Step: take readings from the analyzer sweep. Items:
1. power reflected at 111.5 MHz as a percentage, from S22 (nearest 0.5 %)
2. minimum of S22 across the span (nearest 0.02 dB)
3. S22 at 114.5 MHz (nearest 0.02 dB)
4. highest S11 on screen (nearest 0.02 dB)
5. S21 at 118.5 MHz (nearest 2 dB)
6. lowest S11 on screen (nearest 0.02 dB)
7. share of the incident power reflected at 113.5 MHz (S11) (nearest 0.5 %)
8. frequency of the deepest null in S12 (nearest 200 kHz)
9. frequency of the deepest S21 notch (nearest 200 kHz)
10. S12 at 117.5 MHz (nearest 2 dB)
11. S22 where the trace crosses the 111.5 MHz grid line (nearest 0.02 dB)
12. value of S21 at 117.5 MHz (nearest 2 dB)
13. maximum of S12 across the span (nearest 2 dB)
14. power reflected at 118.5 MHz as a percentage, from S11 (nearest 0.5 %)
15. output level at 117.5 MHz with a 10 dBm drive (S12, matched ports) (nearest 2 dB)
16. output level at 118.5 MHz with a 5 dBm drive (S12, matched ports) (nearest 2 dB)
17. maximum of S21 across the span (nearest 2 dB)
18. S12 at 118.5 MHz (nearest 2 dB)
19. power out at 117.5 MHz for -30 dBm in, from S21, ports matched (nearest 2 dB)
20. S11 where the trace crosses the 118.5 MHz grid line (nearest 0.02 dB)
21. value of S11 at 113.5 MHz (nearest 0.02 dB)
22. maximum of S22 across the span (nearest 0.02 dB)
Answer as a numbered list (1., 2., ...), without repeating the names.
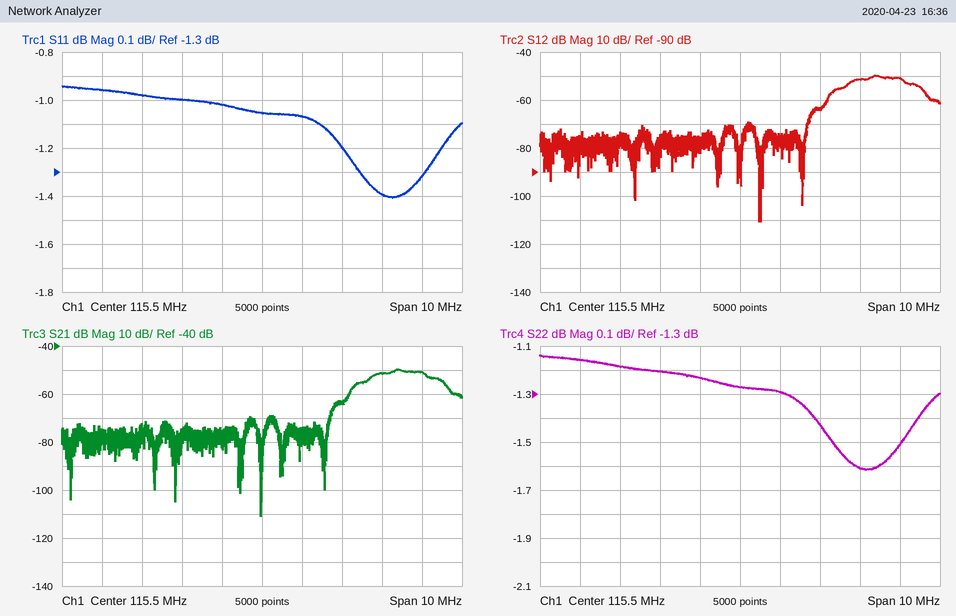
1. 76.5 %
2. -1.62 dB
3. -1.24 dB
4. -0.94 dB
5. -52 dB
6. -1.40 dB
7. 79.5 %
8. 116.0 MHz
9. 115.4 MHz
10. -64 dB
11. -1.16 dB
12. -64 dB
13. -50 dB
14. 72.5 %
15. -54 dBm
16. -46 dBm
17. -50 dB
18. -52 dB
19. -94 dBm
20. -1.40 dB
21. -1.00 dB
22. -1.14 dB
